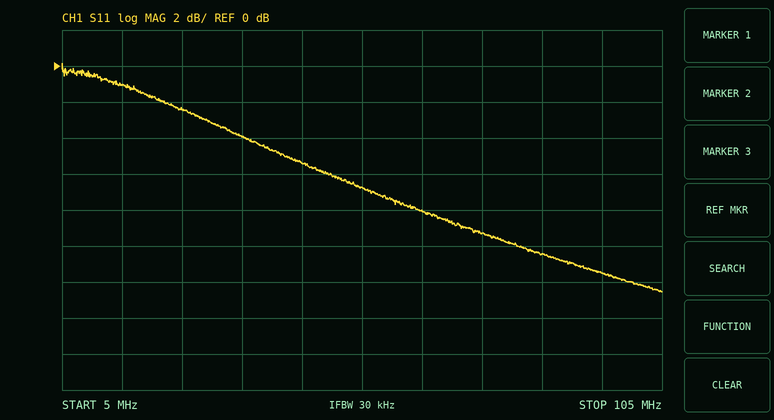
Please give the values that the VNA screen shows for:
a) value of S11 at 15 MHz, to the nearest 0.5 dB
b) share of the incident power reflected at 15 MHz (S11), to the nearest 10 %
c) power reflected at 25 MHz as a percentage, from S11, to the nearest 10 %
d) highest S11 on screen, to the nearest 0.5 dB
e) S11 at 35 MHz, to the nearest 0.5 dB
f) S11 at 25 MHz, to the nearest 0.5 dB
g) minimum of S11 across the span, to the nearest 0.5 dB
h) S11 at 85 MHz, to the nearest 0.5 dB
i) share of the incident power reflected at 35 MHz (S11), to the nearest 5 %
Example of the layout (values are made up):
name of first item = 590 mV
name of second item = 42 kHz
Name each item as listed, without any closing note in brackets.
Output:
value of S11 at 15 MHz, to the nearest 0.5 dB = -1.0 dB
share of the incident power reflected at 15 MHz (S11), to the nearest 10 % = 80 %
power reflected at 25 MHz as a percentage, from S11, to the nearest 10 % = 60 %
highest S11 on screen, to the nearest 0.5 dB = 0.0 dB
S11 at 35 MHz, to the nearest 0.5 dB = -4.0 dB
S11 at 25 MHz, to the nearest 0.5 dB = -2.5 dB
minimum of S11 across the span, to the nearest 0.5 dB = -12.5 dB
S11 at 85 MHz, to the nearest 0.5 dB = -10.5 dB
share of the incident power reflected at 35 MHz (S11), to the nearest 5 % = 40 %
